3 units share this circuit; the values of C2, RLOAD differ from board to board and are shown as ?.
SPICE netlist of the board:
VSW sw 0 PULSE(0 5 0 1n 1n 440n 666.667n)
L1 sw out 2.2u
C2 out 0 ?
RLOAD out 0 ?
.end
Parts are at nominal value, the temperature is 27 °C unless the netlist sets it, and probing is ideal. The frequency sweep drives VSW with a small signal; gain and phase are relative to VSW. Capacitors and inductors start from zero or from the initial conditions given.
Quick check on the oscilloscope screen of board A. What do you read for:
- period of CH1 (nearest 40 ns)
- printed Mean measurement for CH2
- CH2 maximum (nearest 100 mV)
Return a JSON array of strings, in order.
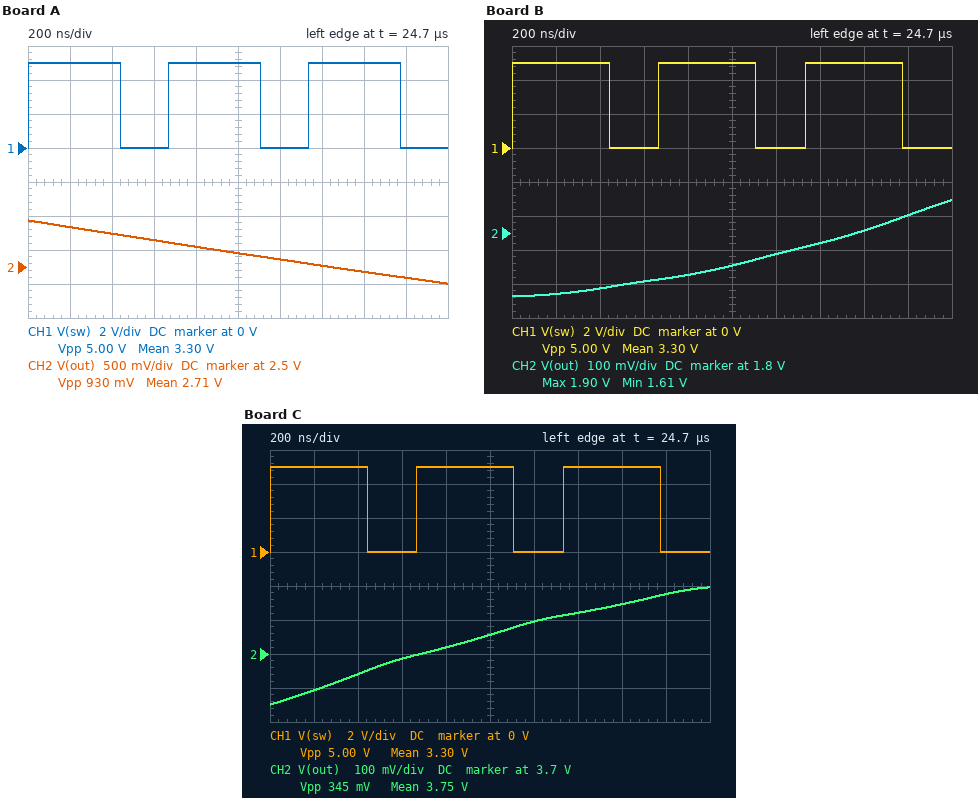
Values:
["680 ns", "2.71 V", "3.2 V"]
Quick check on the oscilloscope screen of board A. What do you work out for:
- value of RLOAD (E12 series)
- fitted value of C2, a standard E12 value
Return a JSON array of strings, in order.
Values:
["3.9 Ω", "12 µF"]
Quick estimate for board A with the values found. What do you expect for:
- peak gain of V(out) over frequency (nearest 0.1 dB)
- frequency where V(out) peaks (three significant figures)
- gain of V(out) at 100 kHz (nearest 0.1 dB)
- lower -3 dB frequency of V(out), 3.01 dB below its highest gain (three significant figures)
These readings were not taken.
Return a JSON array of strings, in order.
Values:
["19.2 dB", "30.9 kHz", "-19.5 dB", "29.1 kHz"]
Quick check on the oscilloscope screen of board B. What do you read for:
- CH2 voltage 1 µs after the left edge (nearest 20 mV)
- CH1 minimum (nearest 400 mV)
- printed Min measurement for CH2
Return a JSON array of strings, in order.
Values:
["1.70 V", "0 V", "1.61 V"]
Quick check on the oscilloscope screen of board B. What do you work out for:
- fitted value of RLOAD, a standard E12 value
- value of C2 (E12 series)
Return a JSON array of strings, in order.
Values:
["2.7 Ω", "6.8 µF"]
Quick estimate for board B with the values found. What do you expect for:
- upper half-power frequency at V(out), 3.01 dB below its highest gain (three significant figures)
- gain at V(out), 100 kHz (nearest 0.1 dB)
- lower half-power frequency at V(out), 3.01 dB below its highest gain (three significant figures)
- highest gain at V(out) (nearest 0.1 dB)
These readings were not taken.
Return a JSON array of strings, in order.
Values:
["44.8 kHz", "-13.9 dB", "36.1 kHz", "13.6 dB"]
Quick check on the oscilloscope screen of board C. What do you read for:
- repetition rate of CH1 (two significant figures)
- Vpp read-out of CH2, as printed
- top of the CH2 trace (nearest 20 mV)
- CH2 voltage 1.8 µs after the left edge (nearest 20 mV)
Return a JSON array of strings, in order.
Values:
["1.5 MHz", "345 mV", "3.90 V", "3.88 V"]
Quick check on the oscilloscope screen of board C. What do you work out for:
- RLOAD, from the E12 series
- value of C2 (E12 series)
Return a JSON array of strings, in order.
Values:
["2.2 Ω", "3.9 µF"]
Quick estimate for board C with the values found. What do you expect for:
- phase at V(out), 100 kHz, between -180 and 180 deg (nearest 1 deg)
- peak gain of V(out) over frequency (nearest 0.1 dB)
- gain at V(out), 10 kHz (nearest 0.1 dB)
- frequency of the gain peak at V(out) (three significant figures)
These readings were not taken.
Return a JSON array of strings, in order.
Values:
["-165 deg", "9.5 dB", "0.3 dB", "52.7 kHz"]
